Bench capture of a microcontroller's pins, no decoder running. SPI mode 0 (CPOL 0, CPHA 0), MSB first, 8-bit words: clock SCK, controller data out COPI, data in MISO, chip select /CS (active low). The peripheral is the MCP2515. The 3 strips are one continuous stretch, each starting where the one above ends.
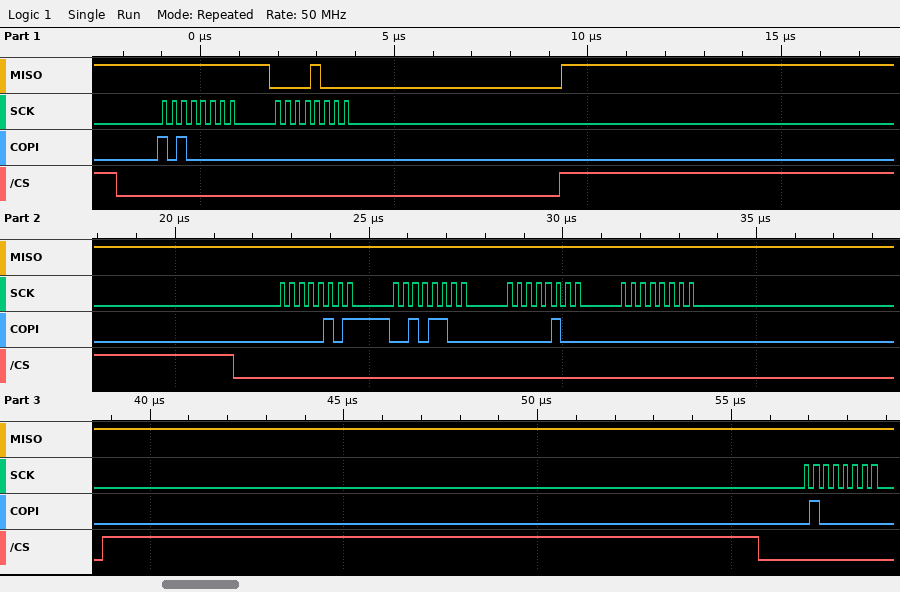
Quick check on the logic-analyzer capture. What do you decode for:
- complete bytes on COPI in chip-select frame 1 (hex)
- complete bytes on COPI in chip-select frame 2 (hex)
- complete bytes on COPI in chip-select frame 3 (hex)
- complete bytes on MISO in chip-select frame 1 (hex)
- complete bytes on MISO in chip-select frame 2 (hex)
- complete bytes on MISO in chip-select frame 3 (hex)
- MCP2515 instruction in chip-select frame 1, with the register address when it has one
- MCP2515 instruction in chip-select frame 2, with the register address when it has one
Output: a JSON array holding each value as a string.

["A0 00", "05 2C 04 00", "40", "FF 08", "FF FF FF FF", "FF", "READ STATUS", "BIT MODIFY 0x2C"]
